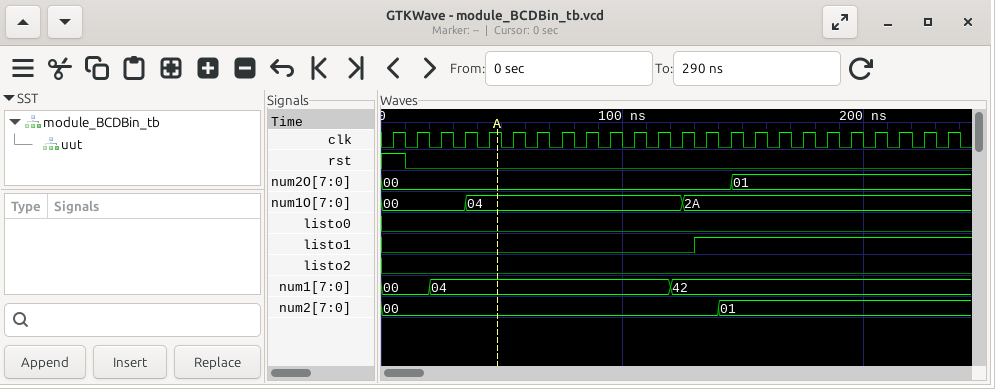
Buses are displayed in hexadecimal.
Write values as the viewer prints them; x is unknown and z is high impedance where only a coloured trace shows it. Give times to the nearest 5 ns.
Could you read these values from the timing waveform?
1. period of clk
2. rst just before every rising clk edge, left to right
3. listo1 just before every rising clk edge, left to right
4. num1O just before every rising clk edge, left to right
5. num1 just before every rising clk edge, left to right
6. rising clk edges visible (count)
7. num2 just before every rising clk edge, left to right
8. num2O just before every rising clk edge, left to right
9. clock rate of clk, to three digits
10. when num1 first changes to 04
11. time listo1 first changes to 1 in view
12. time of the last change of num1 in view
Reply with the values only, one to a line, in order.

10 ns
1 0 0 0 0 0 0 0 0 0 0 0 0 0 0 0 0 0 0 0 0 0 0 0
0 0 0 0 0 0 0 0 0 0 0 0 0 1 1 1 1 1 1 1 1 1 1 1
00, 00, 00, 00, 04, 04, 04, 04, 04, 04, 04, 04, 04, 2A, 2A, 2A, 2A, 2A, 2A, 2A, 2A, 2A, 2A, 2A
00, 00, 04, 04, 04, 04, 04, 04, 04, 04, 04, 04, 42, 42, 42, 42, 42, 42, 42, 42, 42, 42, 42, 42
24
00, 00, 00, 00, 00, 00, 00, 00, 00, 00, 00, 00, 00, 00, 01, 01, 01, 01, 01, 01, 01, 01, 01, 01
00, 00, 00, 00, 00, 00, 00, 00, 00, 00, 00, 00, 00, 00, 00, 01, 01, 01, 01, 01, 01, 01, 01, 01
100 MHz
20 ns
130 ns
120 ns
